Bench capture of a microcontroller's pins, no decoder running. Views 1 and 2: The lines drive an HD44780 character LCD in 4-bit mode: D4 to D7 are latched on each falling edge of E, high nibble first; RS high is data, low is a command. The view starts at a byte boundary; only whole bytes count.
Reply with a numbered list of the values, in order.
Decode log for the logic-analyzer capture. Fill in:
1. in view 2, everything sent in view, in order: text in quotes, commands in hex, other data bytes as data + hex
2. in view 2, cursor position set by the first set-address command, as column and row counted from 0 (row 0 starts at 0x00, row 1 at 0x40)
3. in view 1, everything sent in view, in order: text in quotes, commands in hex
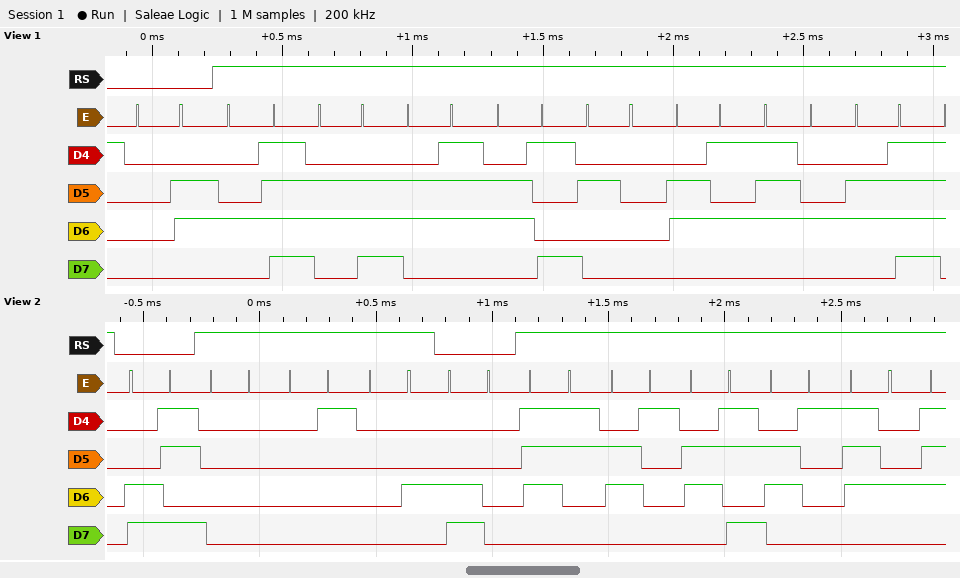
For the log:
1. 0xCB data 00 01 04 0xC0 "sakat"
2. column 11, row 1
3. 0x06 "Ongi eto"
